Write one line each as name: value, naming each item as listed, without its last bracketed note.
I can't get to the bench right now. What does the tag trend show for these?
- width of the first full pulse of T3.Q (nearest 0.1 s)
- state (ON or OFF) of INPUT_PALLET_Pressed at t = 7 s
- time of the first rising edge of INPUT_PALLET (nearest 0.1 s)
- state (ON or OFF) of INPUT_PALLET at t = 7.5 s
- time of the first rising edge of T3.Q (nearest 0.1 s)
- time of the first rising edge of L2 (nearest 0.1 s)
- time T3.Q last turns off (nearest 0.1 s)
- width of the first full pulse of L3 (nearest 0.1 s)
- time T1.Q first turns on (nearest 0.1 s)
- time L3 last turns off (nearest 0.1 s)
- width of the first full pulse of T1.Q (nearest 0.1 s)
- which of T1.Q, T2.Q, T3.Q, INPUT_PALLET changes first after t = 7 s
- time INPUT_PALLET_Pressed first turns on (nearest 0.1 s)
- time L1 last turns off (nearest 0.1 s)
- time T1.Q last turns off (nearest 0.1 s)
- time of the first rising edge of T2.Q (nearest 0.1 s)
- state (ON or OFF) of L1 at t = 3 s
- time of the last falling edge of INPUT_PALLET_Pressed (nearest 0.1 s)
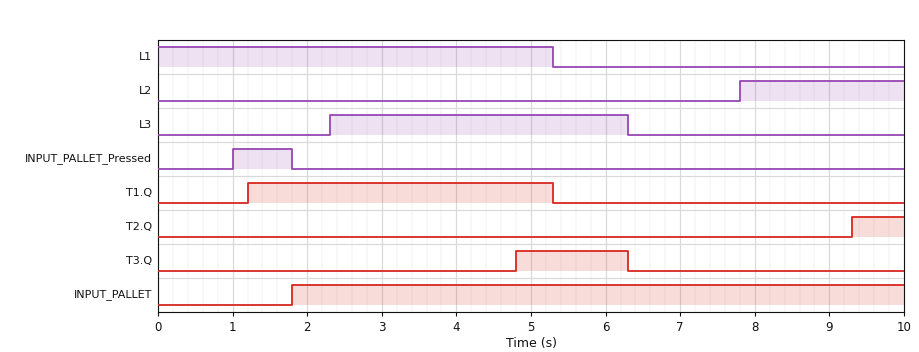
width of the first full pulse of T3.Q: 1.5 s
state (ON or OFF) of INPUT_PALLET_Pressed at t = 7 s: OFF
time of the first rising edge of INPUT_PALLET: 1.8 s
state (ON or OFF) of INPUT_PALLET at t = 7.5 s: ON
time of the first rising edge of T3.Q: 4.8 s
time of the first rising edge of L2: 7.8 s
time T3.Q last turns off: 6.3 s
width of the first full pulse of L3: 4.0 s
time T1.Q first turns on: 1.2 s
time L3 last turns off: 6.3 s
width of the first full pulse of T1.Q: 4.1 s
which of T1.Q, T2.Q, T3.Q, INPUT_PALLET changes first after t = 7 s: T2.Q
time INPUT_PALLET_Pressed first turns on: 1.0 s
time L1 last turns off: 5.3 s
time T1.Q last turns off: 5.3 s
time of the first rising edge of T2.Q: 9.3 s
state (ON or OFF) of L1 at t = 3 s: ON
time of the last falling edge of INPUT_PALLET_Pressed: 1.8 s
